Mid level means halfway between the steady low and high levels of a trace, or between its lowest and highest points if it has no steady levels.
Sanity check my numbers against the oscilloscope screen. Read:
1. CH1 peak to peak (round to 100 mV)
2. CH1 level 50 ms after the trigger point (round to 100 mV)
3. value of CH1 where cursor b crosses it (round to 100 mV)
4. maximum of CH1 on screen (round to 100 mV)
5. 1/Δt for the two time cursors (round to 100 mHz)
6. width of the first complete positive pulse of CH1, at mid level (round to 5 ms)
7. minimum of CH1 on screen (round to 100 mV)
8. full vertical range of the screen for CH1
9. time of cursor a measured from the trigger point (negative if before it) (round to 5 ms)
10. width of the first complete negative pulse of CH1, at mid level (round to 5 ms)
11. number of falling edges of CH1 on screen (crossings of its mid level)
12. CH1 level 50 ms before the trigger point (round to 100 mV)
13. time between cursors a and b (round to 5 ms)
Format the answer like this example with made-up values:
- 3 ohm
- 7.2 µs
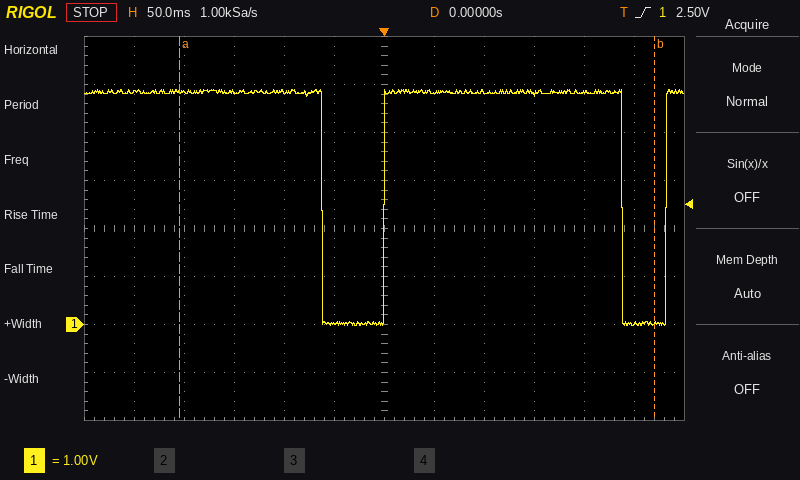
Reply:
- 4.9 V
- 4.8 V
- 0.0 V
- 4.9 V
- 2.1 Hz
- 240 ms
- 0.0 V
- 8 V
- -205 ms
- 60 ms
- 2
- 0.0 V
- 475 ms
